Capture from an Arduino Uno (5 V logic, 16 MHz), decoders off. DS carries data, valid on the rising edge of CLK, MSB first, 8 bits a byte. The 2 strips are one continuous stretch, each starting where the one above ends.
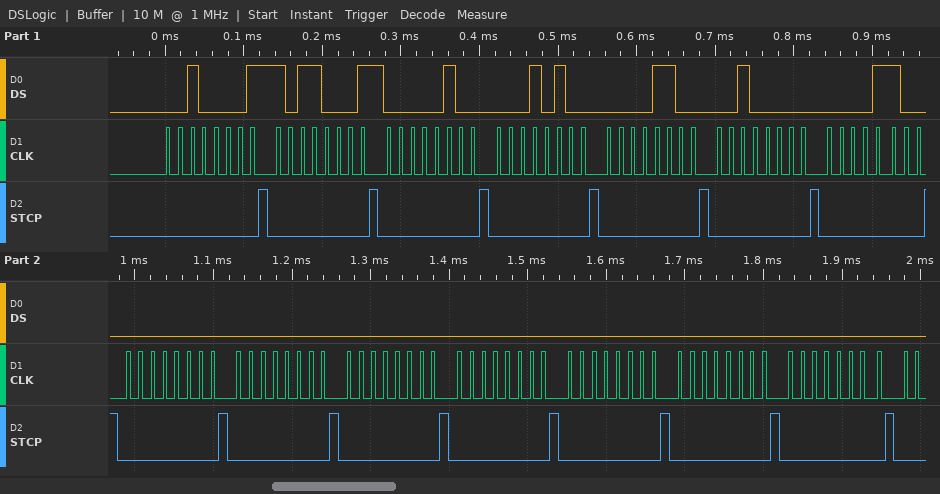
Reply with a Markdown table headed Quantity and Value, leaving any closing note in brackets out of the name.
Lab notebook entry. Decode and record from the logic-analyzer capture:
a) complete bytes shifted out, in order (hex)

| Quantity | Value |
|---|---|
| complete bytes shifted out, in order | 21 B1 04 14 0C 20 0C 00 00 00 00 00 00 00 |
